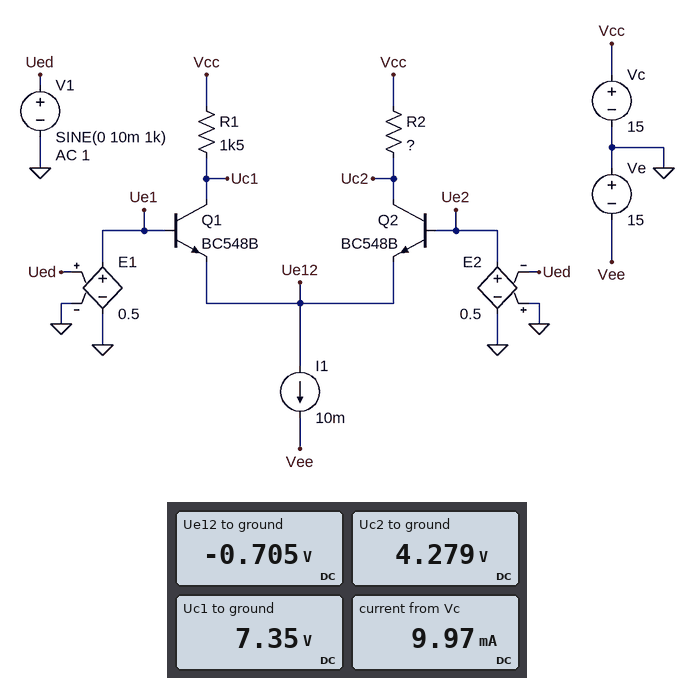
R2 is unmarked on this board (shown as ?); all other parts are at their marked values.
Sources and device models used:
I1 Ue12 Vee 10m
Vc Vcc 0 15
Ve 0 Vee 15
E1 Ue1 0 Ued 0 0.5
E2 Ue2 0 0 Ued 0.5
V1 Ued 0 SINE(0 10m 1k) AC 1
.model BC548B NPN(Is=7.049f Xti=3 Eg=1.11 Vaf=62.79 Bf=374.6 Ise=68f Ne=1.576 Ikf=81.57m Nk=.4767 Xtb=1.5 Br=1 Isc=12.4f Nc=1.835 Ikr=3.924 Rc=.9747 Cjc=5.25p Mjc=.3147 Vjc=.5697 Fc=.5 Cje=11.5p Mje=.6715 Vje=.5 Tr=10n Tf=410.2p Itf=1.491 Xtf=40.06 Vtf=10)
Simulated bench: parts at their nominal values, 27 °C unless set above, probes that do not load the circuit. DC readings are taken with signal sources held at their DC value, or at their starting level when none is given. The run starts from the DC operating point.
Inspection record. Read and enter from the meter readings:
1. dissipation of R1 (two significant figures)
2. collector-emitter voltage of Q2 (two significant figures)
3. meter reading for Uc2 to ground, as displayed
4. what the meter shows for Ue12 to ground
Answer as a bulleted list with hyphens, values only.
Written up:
- 39 mW
- 5.0 V
- 4.279 V
- -0.705 V
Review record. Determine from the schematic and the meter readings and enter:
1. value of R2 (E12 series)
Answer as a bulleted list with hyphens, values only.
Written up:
- 2.2 kΩ
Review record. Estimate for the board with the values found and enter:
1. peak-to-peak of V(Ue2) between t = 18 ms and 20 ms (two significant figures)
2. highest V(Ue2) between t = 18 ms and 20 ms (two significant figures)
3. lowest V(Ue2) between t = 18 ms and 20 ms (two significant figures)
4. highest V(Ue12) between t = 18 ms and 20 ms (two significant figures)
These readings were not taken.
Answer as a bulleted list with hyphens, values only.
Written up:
- 10 mV
- 5.0 mV
- -5.0 mV
- -700 mV
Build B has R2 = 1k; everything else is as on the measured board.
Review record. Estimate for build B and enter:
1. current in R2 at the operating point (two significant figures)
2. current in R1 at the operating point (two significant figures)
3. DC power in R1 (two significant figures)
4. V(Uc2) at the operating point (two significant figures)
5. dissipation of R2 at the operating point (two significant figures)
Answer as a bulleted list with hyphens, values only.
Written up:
- 5.1 mA
- 4.9 mA
- 36 mW
- 9.9 V
- 26 mW
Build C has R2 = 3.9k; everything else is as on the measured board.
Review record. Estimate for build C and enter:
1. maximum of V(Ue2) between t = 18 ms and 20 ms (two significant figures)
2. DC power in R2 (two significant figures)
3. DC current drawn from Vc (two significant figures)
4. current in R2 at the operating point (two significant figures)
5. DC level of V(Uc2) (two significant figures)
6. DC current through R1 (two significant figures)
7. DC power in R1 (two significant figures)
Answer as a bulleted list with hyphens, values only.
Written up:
- 5.0 mV
- 63 mW
- 9.5 mA
- 4.0 mA
- -640 mV
- 5.5 mA
- 45 mW
